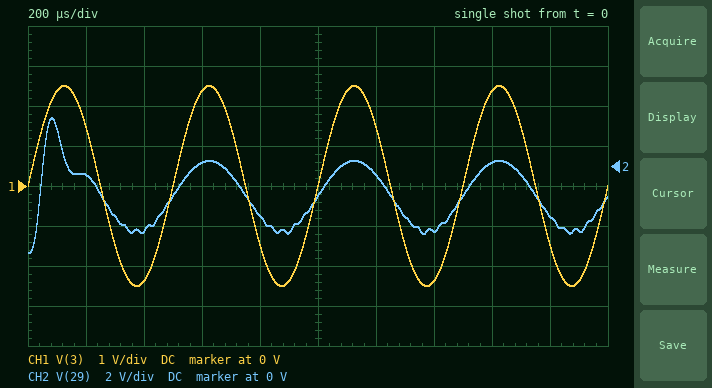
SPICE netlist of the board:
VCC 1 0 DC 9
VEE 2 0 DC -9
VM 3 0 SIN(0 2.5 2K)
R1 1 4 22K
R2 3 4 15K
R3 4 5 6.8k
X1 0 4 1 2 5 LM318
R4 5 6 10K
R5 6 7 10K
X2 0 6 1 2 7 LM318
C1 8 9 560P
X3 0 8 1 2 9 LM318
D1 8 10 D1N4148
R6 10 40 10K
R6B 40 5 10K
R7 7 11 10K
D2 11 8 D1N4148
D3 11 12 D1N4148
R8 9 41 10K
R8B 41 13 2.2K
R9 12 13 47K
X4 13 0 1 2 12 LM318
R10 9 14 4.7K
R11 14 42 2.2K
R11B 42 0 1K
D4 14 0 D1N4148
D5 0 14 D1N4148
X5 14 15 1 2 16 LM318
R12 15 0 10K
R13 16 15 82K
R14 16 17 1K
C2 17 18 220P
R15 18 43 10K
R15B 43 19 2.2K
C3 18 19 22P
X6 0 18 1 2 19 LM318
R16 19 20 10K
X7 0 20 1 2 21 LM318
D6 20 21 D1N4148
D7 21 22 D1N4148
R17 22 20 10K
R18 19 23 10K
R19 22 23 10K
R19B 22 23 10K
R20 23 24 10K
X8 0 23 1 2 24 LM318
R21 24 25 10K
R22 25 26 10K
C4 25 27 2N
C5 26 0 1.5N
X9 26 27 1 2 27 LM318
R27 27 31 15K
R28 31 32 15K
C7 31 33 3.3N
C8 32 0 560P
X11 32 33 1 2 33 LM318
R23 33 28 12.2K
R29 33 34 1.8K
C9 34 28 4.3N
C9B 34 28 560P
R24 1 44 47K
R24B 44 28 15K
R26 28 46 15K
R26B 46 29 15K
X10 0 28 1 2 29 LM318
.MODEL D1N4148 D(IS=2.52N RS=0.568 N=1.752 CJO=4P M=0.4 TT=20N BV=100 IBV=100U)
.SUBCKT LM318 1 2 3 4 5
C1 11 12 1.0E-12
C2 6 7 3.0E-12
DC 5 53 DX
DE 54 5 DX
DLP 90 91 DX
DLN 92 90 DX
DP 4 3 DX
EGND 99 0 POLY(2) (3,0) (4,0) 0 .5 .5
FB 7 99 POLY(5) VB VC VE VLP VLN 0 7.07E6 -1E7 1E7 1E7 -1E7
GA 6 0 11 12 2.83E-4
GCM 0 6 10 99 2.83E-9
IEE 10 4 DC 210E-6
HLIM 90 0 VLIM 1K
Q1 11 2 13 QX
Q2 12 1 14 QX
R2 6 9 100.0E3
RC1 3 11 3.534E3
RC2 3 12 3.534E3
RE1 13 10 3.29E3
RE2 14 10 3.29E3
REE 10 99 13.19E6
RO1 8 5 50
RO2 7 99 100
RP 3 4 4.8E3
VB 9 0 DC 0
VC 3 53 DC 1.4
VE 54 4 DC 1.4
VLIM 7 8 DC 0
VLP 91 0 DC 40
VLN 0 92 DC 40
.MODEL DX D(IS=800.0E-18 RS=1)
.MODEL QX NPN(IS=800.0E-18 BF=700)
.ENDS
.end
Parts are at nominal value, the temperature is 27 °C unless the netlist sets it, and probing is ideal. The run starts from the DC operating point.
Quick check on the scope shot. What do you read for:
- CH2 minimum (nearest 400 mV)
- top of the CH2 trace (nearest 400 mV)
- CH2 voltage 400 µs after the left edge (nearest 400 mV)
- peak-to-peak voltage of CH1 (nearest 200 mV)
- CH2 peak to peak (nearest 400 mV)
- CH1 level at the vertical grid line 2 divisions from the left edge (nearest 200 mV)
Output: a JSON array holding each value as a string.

["-4.4 V", "2.4 V", "-3.2 V", "5.0 V", "6.8 V", "-2.4 V"]
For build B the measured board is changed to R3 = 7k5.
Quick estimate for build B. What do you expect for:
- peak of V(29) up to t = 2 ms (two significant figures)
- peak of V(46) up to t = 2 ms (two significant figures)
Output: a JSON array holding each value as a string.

["3.2 V", "1.6 V"]
